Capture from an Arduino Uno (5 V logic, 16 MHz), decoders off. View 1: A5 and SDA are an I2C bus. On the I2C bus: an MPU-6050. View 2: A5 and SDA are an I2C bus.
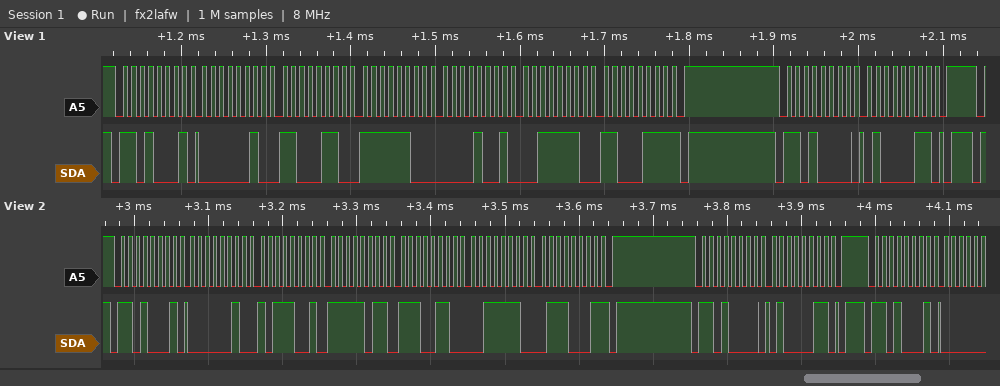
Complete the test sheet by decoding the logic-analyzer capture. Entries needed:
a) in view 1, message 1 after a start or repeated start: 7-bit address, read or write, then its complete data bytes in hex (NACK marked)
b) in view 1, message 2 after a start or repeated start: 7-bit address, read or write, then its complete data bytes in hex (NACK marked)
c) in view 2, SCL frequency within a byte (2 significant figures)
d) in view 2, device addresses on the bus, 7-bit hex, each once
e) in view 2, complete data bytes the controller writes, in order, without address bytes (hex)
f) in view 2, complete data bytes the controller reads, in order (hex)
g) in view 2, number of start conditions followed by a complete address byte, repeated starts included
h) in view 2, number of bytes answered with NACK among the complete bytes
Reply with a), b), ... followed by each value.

a) 0x68 read: 02 C6 FC 09 3E C7 NACK
b) 0x68 write: 43
c) 100 kHz
d) 0x68
e) 43
f) 02 B9 FB E6 3E 71
g) 3
h) 1
